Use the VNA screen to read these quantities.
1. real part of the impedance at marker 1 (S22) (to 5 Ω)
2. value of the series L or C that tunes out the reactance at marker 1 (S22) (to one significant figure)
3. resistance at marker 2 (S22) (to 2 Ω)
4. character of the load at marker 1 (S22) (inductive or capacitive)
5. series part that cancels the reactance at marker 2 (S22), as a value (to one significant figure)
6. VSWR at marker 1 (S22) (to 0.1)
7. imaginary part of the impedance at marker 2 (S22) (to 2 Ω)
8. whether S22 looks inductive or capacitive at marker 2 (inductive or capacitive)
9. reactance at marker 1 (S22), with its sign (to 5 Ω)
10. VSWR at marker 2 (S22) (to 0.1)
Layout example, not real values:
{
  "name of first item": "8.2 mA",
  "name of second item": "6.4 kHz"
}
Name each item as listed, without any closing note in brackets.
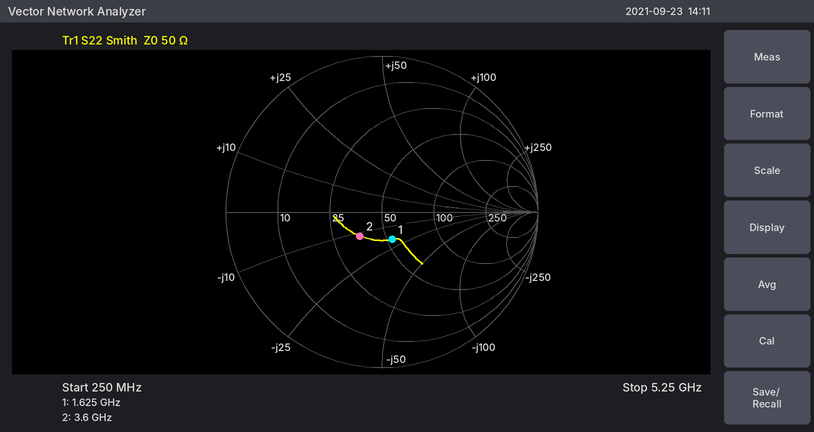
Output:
{
  "real part of the impedance at marker 1 (S22)": "55 Ω",
  "value of the series L or C that tunes out the reactance at marker 1 (S22)": "2 nH",
  "resistance at marker 2 (S22)": "36 Ω",
  "character of the load at marker 1 (S22)": "capacitive",
  "series part that cancels the reactance at marker 2 (S22), as a value": "500 pH",
  "VSWR at marker 1 (S22)": "1.5",
  "imaginary part of the impedance at marker 2 (S22)": "-12 Ω",
  "whether S22 looks inductive or capacitive at marker 2": "capacitive",
  "reactance at marker 1 (S22), with its sign": "-20 Ω",
  "VSWR at marker 2 (S22)": "1.5"
}
